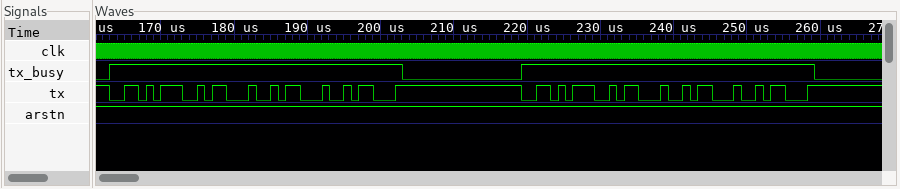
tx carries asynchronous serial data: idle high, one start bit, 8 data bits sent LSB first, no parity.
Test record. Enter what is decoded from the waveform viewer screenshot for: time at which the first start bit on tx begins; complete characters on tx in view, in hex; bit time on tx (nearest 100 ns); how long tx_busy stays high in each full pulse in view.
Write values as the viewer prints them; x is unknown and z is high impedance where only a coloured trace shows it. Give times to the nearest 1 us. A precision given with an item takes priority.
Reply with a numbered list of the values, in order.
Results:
1. 163 us
2. D6, 1A, 1A, 1A, D6, 1A, 1A, 1A
3. 1000 ns
4. 40 us, 40 us
